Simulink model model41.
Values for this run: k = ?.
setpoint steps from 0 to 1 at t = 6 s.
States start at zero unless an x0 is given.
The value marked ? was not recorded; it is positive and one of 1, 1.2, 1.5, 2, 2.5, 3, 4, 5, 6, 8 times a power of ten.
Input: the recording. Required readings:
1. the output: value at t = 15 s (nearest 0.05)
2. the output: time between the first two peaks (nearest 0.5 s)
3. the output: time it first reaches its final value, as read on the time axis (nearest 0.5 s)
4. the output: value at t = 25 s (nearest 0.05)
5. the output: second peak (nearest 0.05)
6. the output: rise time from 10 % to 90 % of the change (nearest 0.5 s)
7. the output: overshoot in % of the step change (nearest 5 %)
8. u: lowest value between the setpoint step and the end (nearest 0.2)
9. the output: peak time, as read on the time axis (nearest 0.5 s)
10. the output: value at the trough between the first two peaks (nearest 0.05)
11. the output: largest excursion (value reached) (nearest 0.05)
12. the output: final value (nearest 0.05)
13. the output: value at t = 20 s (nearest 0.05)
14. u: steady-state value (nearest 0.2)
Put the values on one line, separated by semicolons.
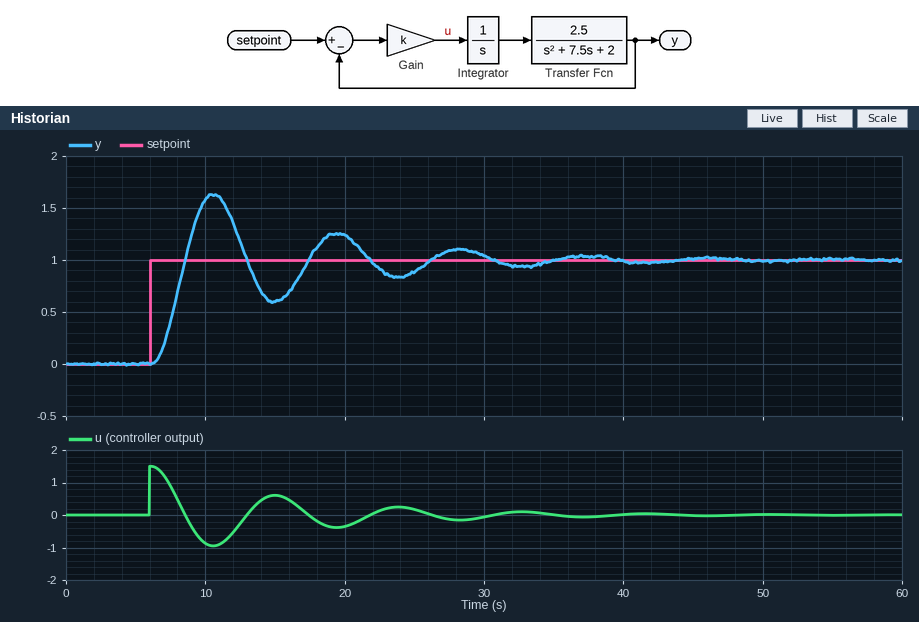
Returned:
0.60; 9.0 s; 8.5 s; 0.90; 1.25; 1.5 s; 65 %; -1.0; 10.5 s; 0.60; 1.65; 1.00; 1.25; 0.0
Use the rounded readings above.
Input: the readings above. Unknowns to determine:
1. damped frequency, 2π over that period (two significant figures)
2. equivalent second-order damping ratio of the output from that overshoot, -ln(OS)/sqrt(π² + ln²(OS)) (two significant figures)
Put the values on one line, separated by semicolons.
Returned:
0.70 rad/s; 0.14
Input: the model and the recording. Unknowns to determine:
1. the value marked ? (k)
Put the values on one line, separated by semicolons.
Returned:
1.5
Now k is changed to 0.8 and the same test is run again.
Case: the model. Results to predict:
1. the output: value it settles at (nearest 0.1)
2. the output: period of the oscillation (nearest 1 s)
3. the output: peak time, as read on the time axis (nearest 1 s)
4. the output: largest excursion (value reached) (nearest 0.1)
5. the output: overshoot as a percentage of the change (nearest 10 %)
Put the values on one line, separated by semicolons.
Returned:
1.0; 12 s; 12 s; 1.5; 50 %
